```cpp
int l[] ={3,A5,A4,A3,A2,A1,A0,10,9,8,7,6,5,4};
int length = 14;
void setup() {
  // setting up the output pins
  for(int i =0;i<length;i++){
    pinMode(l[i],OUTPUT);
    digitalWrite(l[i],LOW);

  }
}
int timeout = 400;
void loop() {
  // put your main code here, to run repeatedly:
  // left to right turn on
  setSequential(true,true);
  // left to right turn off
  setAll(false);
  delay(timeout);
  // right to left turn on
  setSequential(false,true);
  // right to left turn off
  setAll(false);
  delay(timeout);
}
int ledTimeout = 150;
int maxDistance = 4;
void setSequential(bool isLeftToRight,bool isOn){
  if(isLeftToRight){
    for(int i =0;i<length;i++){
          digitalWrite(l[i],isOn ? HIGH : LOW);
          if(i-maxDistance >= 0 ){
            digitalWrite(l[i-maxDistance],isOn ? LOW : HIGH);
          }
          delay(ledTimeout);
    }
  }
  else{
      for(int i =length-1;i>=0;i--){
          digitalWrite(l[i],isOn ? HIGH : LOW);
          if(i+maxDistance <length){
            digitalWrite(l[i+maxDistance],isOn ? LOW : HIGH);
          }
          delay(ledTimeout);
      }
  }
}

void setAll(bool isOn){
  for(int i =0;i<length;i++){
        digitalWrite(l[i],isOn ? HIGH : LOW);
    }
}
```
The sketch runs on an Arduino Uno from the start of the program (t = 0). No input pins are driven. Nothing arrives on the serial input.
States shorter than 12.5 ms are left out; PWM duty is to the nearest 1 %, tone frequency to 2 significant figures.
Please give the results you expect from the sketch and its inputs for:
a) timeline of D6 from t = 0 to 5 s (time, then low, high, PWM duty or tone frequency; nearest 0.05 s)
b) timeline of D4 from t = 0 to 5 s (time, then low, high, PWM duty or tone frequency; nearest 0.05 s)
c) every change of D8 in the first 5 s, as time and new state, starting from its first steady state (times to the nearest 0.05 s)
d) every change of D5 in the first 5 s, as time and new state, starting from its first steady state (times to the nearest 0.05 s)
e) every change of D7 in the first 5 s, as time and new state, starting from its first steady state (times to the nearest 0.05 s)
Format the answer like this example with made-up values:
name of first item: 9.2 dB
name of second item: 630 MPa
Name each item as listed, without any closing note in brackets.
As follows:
timeline of D6 from t = 0 to 5 s: 0 s low; 1.65 s high; 2.1 s low; 2.8 s high; 3.4 s low
timeline of D4 from t = 0 to 5 s: 0 s low; 1.95 s high; 2.1 s low; 2.5 s high; 3.1 s low
every change of D8 in the first 5 s, as time and new state, starting from its first steady state: 0 s low; 1.35 s high; 1.95 s low; 3.1 s high; 3.7 s low
every change of D5 in the first 5 s, as time and new state, starting from its first steady state: 0 s low; 1.8 s high; 2.1 s low; 2.65 s high; 3.25 s low
every change of D7 in the first 5 s, as time and new state, starting from its first steady state: 0 s low; 1.5 s high; 2.1 s low; 2.95 s high; 3.55 s low
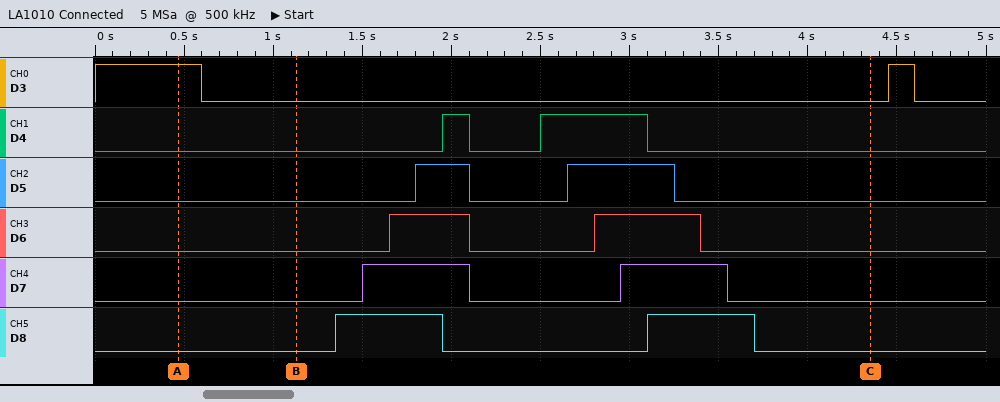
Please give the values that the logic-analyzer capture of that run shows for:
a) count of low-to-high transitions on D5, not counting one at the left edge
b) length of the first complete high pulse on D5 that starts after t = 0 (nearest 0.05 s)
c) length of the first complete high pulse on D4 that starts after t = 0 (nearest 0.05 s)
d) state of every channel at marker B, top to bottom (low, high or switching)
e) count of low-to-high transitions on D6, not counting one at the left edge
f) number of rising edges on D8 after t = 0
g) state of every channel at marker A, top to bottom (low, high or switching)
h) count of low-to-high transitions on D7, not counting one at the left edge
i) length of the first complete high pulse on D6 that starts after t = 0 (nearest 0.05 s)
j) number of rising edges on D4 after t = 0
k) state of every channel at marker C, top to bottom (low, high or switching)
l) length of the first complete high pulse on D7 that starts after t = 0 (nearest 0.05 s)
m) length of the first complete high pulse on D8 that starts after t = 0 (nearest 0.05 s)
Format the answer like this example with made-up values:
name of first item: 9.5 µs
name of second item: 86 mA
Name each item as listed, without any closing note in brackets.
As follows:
count of low-to-high transitions on D5, not counting one at the left edge: 2
length of the first complete high pulse on D5 that starts after t = 0: 0.30 s
length of the first complete high pulse on D4 that starts after t = 0: 0.15 s
state of every channel at marker B, top to bottom: D3 low, D4 low, D5 low, D6 low, D7 low, D8 low
count of low-to-high transitions on D6, not counting one at the left edge: 2
number of rising edges on D8 after t = 0: 2
state of every channel at marker A, top to bottom: D3 high, D4 low, D5 low, D6 low, D7 low, D8 low
count of low-to-high transitions on D7, not counting one at the left edge: 2
length of the first complete high pulse on D6 that starts after t = 0: 0.45 s
number of rising edges on D4 after t = 0: 2
state of every channel at marker C, top to bottom: D3 low, D4 low, D5 low, D6 low, D7 low, D8 low
length of the first complete high pulse on D7 that starts after t = 0: 0.60 s
length of the first complete high pulse on D8 that starts after t = 0: 0.60 s
